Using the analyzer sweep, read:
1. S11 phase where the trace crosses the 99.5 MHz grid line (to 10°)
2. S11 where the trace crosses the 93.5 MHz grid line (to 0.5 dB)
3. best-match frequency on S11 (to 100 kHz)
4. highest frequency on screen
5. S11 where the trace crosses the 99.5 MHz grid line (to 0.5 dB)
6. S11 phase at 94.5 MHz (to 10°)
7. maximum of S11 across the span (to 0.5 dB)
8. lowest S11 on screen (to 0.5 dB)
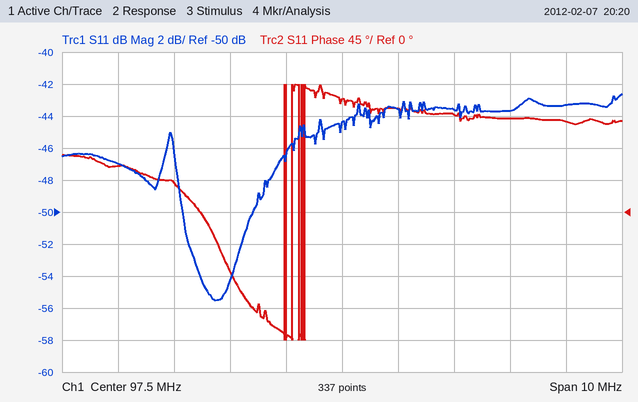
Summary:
140°
-47.0 dB
95.2 MHz
102.5 MHz
-43.5 dB
40°
-42.5 dB
-55.5 dB
